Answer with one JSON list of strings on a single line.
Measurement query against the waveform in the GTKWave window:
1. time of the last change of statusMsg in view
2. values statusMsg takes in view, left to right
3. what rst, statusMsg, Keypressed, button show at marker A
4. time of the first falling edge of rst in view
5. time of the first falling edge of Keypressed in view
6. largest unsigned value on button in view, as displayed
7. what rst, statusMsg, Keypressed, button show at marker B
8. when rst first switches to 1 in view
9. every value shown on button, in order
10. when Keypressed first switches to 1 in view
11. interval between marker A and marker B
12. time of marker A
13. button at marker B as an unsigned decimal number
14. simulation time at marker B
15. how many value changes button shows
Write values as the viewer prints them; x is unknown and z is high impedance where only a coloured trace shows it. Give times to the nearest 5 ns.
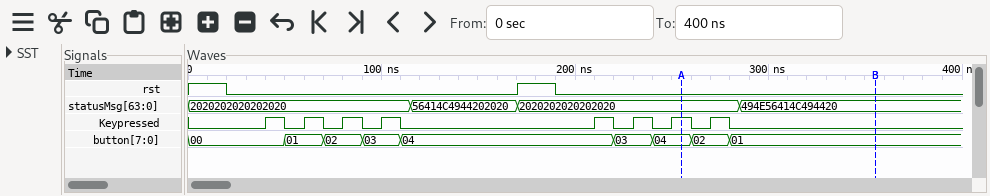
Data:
["285 ns", "2020202020202020, 56414C4944202020, 2020202020202020, 494E56414C494420", "rst=0, statusMsg=2020202020202020, Keypressed=1, button=04", "20 ns", "50 ns", "04", "rst=0, statusMsg=494E56414C494420, Keypressed=0, button=01", "170 ns", "00, 01, 02, 03, 04, 03, 04, 02, 01", "40 ns", "100 ns", "255 ns", "1", "355 ns", "8"]
